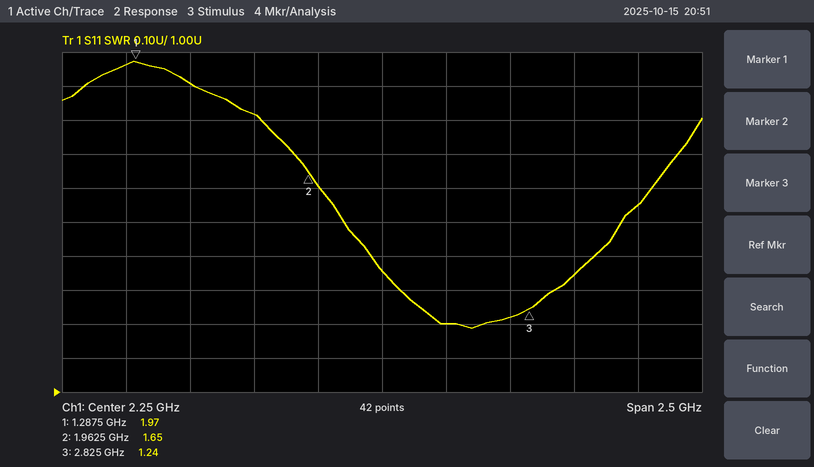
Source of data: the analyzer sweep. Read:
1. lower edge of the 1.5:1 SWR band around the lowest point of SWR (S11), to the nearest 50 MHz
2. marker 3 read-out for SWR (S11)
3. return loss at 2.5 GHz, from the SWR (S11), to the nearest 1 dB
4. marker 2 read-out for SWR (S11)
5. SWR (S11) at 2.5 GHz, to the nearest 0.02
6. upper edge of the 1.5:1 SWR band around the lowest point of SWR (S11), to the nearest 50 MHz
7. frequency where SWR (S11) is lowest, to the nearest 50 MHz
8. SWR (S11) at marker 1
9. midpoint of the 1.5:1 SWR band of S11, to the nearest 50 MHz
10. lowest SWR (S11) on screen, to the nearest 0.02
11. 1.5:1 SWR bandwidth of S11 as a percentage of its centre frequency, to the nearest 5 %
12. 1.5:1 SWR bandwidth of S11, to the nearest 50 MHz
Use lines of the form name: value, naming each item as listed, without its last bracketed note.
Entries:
lower edge of the 1.5:1 SWR band around the lowest point of SWR (S11), to the nearest 50 MHz: 2.10 GHz
marker 3 read-out for SWR: 1.24
return loss at 2.5 GHz, from the SWR (S11), to the nearest 1 dB: 21 dB
marker 2 read-out for SWR: 1.65
SWR (S11) at 2.5 GHz, to the nearest 0.02: 1.20
upper edge of the 1.5:1 SWR band around the lowest point of SWR (S11), to the nearest 50 MHz: 3.20 GHz
frequency where SWR (S11) is lowest, to the nearest 50 MHz: 2.60 GHz
SWR (S11) at marker 1: 1.97
midpoint of the 1.5:1 SWR band of S11, to the nearest 50 MHz: 2.65 GHz
lowest SWR (S11) on screen, to the nearest 0.02: 1.18
1.5:1 SWR bandwidth of S11 as a percentage of its centre frequency, to the nearest 5 %: 40 %
1.5:1 SWR bandwidth of S11, to the nearest 50 MHz: 1.10 GHz
